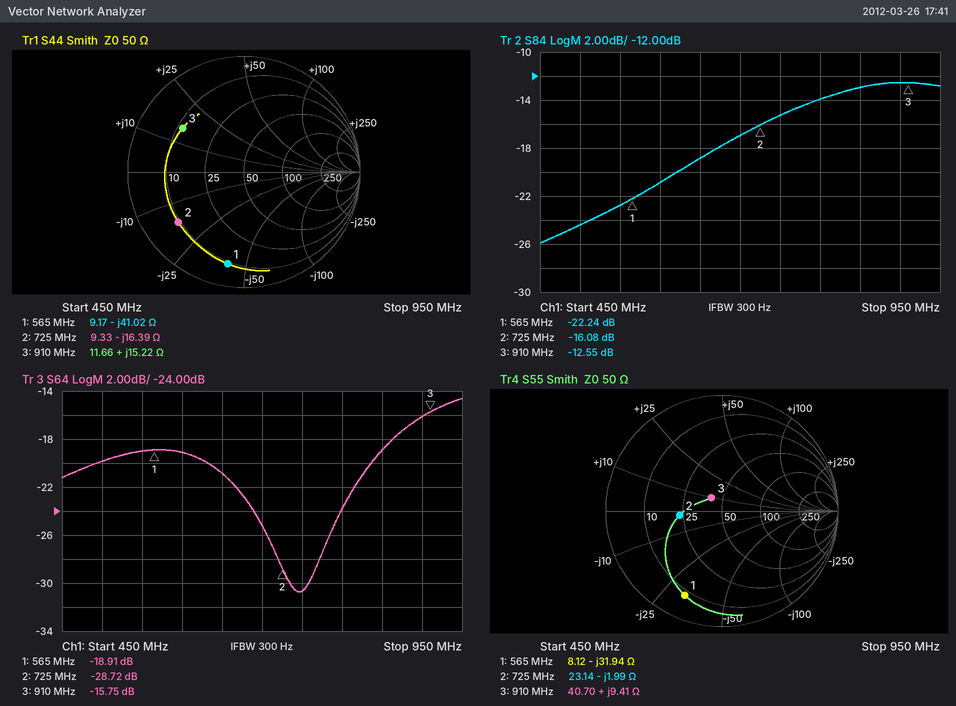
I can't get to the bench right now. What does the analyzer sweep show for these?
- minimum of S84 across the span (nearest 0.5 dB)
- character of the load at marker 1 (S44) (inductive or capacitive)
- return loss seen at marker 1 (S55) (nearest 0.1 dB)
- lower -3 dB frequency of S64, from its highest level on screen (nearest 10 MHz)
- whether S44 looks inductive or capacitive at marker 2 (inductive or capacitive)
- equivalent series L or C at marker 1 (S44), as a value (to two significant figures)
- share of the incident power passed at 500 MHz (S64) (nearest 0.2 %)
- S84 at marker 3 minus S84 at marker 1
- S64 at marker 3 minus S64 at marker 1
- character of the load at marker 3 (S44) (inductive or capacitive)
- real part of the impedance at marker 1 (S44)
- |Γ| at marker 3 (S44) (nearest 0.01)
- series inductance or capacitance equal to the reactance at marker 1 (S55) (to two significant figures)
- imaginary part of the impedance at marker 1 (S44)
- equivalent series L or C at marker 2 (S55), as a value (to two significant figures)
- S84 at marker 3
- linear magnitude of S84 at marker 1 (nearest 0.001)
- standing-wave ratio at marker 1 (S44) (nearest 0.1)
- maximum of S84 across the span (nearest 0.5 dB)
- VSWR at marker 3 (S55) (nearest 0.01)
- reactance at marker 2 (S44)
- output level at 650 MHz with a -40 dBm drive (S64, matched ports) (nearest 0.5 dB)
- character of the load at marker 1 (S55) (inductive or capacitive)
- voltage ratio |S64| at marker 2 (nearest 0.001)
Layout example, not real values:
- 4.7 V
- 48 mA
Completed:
- -26.0 dB
- capacitive
- 2.0 dB
- 870 MHz
- capacitive
- 6.9 pF
- 1.0 %
- 9.69 dB
- 3.16 dB
- inductive
- 9.17 Ω
- 0.65
- 8.8 pF
- -41.02 Ω
- 110 pF
- -12.55 dB
- 0.077
- 9.2
- -12.5 dB
- 1.34
- -16.39 Ω
- -61.0 dBm
- capacitive
- 0.037
